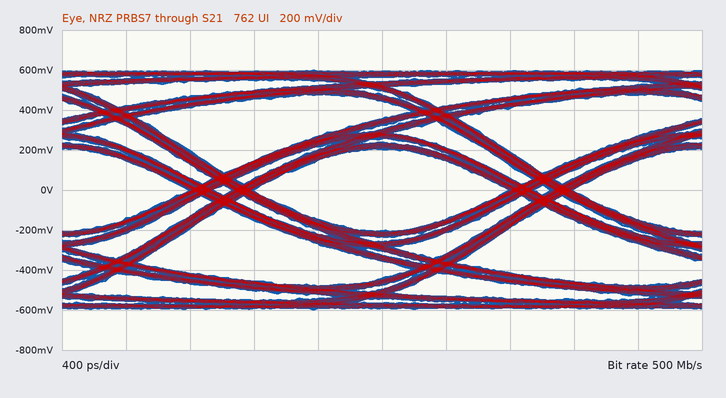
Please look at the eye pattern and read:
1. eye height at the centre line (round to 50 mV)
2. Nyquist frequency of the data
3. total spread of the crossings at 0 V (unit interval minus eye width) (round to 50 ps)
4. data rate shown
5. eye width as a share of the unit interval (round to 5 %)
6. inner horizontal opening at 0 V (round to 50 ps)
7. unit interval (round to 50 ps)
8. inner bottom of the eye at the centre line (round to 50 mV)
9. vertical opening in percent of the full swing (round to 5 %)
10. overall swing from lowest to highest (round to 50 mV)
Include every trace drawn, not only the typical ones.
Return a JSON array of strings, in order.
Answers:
["400 mV", "250 MHz", "400 ps", "500 Mb/s", "80 %", "1.60 ns", "2.00 ns", "-200 mV", "35 %", "1.20 V"]
